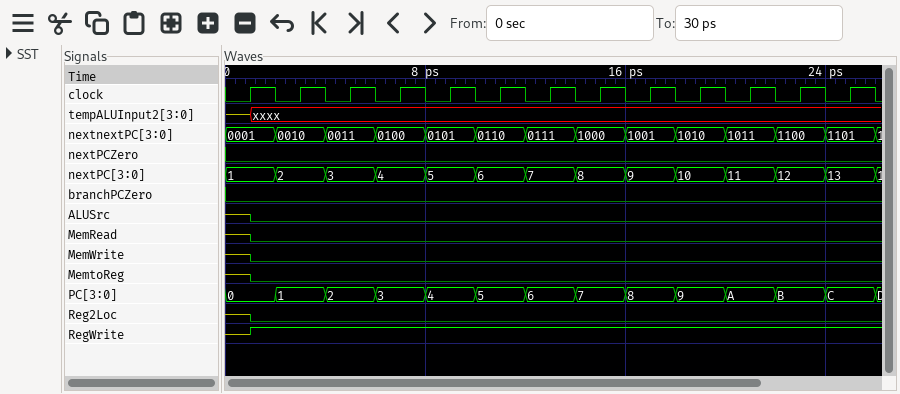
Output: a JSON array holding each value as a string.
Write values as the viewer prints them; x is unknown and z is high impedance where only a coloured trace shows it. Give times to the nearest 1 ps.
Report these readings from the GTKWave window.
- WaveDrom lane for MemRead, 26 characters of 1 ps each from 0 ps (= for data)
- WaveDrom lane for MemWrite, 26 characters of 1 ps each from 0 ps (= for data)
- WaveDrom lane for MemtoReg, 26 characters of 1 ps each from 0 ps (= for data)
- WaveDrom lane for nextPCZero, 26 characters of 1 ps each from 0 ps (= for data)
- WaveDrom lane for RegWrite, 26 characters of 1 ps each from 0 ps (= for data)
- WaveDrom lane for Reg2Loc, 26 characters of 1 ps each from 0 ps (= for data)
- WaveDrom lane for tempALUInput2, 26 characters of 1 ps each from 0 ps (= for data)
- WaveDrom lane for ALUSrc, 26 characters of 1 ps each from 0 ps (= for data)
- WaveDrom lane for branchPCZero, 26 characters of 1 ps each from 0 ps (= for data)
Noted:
["{name: 'MemRead', wave: 'z0........................'}", "{name: 'MemWrite', wave: 'z0........................'}", "{name: 'MemtoReg', wave: 'z0........................'}", "{name: 'nextPCZero', wave: '0.........................'}", "{name: 'RegWrite', wave: 'z1........................'}", "{name: 'Reg2Loc', wave: 'z0........................'}", "{name: 'tempALUInput2', wave: 'zx........................'}", "{name: 'ALUSrc', wave: 'z0........................'}", "{name: 'branchPCZero', wave: '0.........................'}"]
